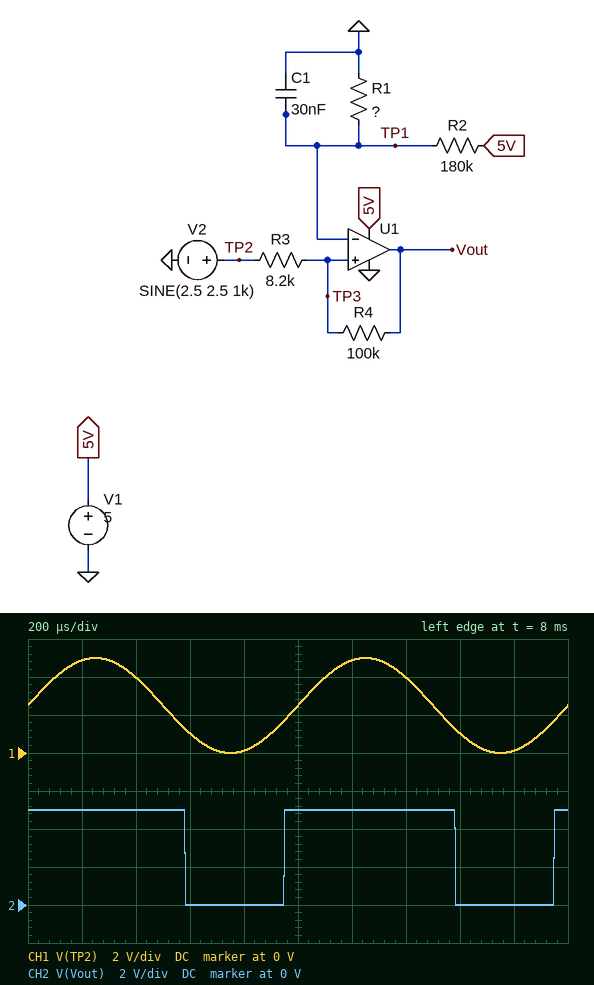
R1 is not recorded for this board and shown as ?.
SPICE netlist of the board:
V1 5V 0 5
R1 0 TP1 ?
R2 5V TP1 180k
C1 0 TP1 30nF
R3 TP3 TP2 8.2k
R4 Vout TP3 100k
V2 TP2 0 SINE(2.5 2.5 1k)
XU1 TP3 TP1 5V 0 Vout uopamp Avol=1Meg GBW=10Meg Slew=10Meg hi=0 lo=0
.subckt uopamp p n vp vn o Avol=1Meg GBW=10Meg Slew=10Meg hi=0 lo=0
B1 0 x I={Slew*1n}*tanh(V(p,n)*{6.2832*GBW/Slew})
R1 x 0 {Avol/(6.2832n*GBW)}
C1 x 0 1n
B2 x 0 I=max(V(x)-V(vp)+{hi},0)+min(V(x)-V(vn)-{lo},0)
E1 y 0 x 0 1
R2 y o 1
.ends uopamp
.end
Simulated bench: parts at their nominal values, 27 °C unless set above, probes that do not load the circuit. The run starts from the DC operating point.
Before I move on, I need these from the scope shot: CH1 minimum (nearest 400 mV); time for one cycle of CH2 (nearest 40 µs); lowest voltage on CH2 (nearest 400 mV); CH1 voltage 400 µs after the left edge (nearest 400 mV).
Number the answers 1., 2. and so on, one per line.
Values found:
1. 0 V
2. 1.00 ms
3. 0 V
4. 4.0 V
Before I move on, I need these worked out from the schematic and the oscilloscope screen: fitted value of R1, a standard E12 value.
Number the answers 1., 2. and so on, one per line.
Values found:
1. 82 kΩ
